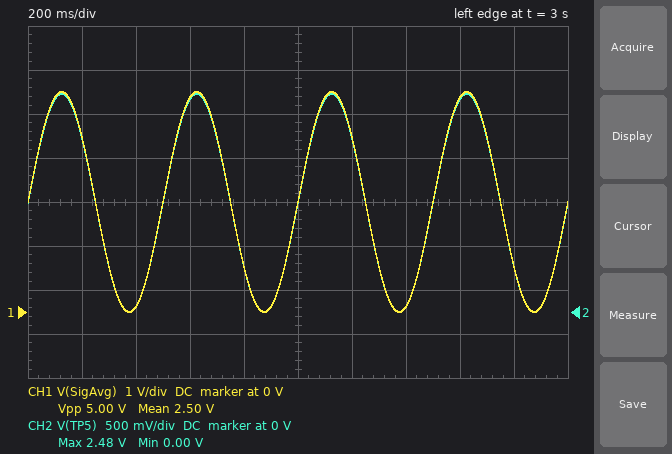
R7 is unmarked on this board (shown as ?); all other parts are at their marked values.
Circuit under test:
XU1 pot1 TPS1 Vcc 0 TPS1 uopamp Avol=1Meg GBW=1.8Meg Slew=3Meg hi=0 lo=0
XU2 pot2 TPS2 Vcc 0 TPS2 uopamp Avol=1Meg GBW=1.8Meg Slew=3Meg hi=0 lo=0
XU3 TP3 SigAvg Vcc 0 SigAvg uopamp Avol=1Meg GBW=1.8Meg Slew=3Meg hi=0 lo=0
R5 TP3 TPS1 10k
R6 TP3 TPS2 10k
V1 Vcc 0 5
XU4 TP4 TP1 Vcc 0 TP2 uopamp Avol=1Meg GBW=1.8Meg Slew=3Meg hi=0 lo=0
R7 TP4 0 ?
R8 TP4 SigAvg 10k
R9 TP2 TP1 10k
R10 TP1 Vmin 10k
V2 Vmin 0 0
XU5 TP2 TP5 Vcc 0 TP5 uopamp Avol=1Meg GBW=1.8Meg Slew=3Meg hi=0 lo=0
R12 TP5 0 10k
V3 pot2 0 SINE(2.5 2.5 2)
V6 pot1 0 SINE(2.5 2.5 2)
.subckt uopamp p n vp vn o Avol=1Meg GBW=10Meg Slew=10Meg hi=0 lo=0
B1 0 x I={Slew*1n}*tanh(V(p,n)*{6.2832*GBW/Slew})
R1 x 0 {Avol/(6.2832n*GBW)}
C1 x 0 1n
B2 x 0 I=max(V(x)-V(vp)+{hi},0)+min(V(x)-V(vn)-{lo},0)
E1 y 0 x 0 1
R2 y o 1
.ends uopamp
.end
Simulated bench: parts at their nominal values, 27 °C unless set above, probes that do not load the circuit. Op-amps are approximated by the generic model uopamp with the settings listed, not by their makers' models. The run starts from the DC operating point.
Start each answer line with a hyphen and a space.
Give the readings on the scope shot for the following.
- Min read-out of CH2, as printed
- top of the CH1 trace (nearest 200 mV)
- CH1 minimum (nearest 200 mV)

- 0.00 V
- 5.0 V
- 0 V
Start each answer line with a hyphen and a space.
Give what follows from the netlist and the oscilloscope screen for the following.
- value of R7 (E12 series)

- 3.3 kΩ
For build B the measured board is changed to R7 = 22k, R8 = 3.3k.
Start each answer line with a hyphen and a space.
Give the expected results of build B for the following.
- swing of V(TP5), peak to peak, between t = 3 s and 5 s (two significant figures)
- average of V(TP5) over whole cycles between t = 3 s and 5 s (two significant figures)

- 5.0 V
- 3.3 V
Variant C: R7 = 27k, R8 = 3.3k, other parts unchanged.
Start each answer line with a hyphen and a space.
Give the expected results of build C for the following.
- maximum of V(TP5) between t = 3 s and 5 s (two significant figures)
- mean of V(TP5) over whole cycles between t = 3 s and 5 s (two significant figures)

- 5.0 V
- 3.3 V
